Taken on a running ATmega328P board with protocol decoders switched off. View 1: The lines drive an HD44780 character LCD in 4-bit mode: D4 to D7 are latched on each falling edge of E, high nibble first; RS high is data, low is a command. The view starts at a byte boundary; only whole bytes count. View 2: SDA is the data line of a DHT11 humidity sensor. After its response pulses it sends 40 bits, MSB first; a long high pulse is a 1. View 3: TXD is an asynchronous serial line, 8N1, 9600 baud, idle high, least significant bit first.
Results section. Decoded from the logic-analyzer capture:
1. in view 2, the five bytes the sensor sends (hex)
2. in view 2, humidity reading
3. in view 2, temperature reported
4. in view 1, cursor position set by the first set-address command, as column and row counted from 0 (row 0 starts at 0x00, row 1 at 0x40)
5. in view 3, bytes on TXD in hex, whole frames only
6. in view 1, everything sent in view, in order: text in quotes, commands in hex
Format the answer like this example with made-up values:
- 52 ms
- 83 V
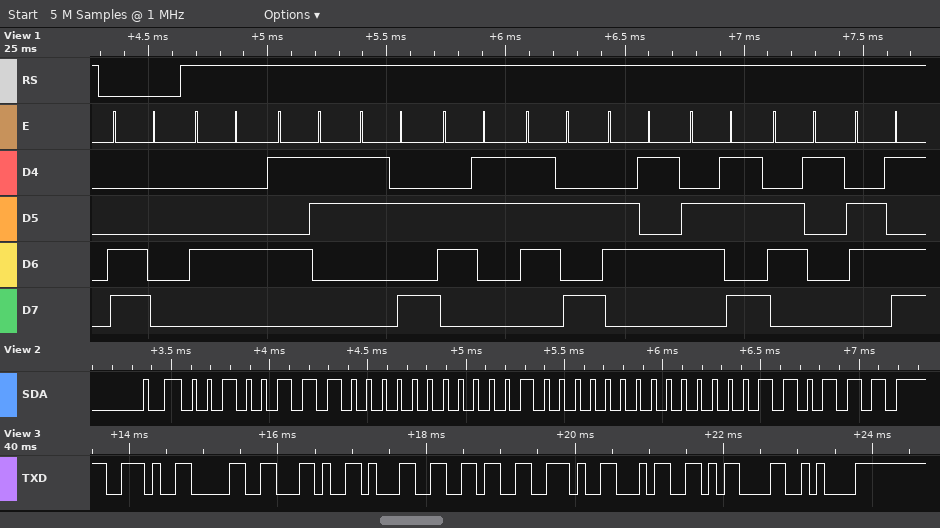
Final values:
- 27 00 10 00 37
- 39 %
- 16.0 °C
- column 0, row 1
- 2E 30 2C 31 36 2E 34 0D 0A
- 0xC0 "DS:czekam"
